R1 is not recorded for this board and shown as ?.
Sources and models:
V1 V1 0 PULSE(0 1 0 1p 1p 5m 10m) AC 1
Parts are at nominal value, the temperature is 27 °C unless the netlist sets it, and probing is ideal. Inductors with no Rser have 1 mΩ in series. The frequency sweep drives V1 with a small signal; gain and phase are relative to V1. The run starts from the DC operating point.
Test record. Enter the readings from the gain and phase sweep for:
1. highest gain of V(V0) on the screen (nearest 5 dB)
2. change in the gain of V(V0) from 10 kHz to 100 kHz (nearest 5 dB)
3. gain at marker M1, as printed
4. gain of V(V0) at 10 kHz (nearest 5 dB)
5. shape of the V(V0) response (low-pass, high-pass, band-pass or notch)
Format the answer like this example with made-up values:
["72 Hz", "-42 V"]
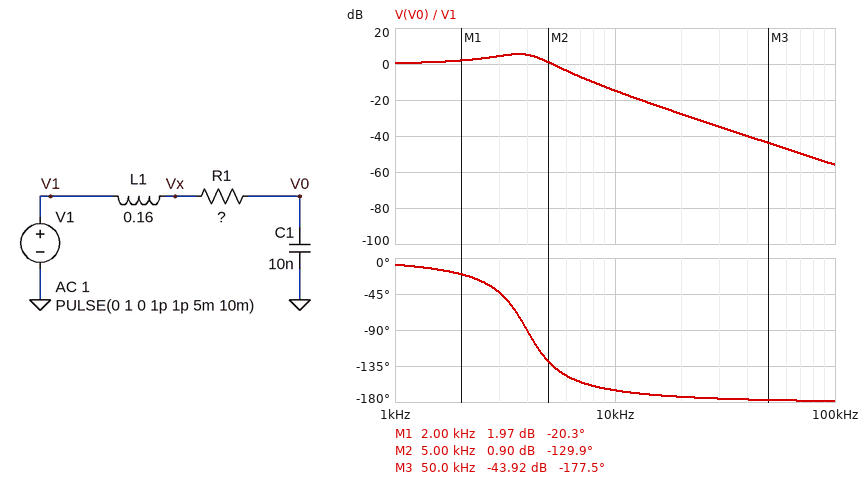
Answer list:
["5 dB", "-40 dB", "1.97 dB", "-15 dB", "low-pass"]
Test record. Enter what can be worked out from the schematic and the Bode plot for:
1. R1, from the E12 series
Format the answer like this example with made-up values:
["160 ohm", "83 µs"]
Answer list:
["2.2 kΩ"]
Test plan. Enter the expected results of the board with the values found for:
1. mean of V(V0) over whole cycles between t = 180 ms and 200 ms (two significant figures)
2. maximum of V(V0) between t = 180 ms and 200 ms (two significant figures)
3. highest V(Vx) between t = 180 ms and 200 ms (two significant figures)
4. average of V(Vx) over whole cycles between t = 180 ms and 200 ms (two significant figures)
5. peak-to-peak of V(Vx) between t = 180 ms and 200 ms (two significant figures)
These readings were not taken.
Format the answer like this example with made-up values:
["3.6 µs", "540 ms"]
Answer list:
["500 mV", "1.4 V", "1.5 V", "500 mV", "2.0 V"]
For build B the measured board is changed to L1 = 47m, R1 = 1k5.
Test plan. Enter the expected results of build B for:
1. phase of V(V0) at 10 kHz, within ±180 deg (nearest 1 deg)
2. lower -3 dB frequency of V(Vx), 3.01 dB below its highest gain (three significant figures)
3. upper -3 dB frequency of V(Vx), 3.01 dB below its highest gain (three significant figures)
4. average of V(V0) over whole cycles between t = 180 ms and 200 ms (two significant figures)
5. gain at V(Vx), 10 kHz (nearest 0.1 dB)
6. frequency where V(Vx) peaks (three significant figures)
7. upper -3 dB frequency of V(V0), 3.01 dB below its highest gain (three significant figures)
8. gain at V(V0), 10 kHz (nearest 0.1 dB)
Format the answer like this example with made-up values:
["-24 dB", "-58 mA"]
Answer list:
["-132 deg", "3.67 kHz", "9.18 kHz", "500 mV", "0.7 dB", "6.70 kHz", "8.72 kHz", "-2.1 dB"]
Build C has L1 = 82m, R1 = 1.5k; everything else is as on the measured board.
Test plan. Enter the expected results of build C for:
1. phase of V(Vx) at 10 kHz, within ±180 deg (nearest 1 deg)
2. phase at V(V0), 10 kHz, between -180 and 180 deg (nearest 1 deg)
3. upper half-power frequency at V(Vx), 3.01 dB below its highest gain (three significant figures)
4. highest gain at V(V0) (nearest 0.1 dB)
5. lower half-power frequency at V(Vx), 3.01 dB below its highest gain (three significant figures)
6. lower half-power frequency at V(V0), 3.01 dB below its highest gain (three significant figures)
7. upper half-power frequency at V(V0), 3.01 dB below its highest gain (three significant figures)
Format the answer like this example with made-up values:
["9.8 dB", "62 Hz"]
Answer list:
["-114 deg", "-157 deg", "6.64 kHz", "5.9 dB", "3.57 kHz", "3.32 kHz", "6.50 kHz"]
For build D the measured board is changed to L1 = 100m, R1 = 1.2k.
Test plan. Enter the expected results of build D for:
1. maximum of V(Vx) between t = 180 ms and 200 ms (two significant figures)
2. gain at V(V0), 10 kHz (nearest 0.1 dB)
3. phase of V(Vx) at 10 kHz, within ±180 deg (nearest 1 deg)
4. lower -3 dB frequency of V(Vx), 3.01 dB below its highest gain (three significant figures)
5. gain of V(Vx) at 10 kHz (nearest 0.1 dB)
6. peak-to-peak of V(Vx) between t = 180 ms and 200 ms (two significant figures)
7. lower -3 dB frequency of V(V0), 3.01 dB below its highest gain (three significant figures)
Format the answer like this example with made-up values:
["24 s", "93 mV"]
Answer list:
["1.6 V", "-9.7 dB", "-129 deg", "3.81 kHz", "-7.7 dB", "2.2 V", "3.75 kHz"]
